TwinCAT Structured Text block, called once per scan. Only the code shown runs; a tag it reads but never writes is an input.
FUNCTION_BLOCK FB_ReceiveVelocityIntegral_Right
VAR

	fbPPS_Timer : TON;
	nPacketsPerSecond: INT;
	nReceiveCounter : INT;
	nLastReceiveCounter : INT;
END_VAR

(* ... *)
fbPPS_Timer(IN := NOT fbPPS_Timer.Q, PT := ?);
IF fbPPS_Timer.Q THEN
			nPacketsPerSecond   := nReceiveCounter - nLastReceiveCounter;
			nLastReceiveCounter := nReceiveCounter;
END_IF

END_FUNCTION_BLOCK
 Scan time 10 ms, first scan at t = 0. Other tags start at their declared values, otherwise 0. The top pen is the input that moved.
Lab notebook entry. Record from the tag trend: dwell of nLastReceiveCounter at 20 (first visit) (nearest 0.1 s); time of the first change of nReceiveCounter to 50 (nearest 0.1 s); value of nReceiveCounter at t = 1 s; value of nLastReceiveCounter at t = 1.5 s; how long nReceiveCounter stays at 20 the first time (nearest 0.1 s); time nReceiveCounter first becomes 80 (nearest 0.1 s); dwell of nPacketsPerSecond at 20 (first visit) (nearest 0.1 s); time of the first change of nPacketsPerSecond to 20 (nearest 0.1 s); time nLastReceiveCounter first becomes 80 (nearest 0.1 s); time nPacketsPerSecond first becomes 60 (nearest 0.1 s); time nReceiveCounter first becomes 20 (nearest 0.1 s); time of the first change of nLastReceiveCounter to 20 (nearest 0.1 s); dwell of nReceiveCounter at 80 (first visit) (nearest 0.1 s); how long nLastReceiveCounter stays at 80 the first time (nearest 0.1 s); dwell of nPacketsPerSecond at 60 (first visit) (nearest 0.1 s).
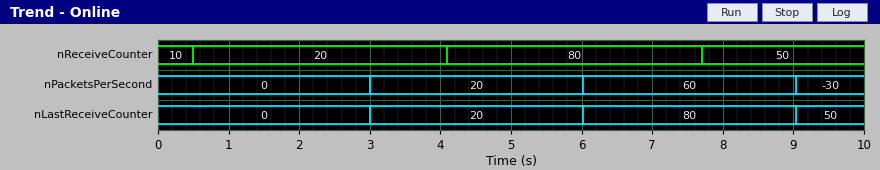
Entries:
3.0 s
7.7 s
20
0
3.6 s
4.1 s
3.0 s
3.0 s
6.0 s
6.0 s
0.5 s
3.0 s
3.6 s
3.0 s
3.0 s
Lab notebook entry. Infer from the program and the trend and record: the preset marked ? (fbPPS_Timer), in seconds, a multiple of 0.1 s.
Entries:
3.0 s
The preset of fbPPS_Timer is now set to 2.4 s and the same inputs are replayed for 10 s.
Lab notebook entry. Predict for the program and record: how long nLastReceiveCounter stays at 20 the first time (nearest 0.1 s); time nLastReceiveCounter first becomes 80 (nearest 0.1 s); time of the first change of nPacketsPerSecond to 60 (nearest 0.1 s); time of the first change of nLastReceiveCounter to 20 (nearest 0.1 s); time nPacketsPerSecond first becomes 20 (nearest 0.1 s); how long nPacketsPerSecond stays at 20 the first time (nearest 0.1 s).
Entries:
2.4 s
4.8 s
4.8 s
2.4 s
2.4 s
2.4 s
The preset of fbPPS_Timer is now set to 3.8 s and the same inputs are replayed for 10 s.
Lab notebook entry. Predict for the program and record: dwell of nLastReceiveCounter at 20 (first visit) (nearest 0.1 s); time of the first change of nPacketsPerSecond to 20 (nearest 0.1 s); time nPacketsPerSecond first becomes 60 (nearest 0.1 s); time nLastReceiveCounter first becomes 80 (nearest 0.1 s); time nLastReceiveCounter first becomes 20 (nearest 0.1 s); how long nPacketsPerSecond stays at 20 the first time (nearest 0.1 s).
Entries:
3.8 s
3.8 s
7.6 s
7.6 s
3.8 s
3.8 s
